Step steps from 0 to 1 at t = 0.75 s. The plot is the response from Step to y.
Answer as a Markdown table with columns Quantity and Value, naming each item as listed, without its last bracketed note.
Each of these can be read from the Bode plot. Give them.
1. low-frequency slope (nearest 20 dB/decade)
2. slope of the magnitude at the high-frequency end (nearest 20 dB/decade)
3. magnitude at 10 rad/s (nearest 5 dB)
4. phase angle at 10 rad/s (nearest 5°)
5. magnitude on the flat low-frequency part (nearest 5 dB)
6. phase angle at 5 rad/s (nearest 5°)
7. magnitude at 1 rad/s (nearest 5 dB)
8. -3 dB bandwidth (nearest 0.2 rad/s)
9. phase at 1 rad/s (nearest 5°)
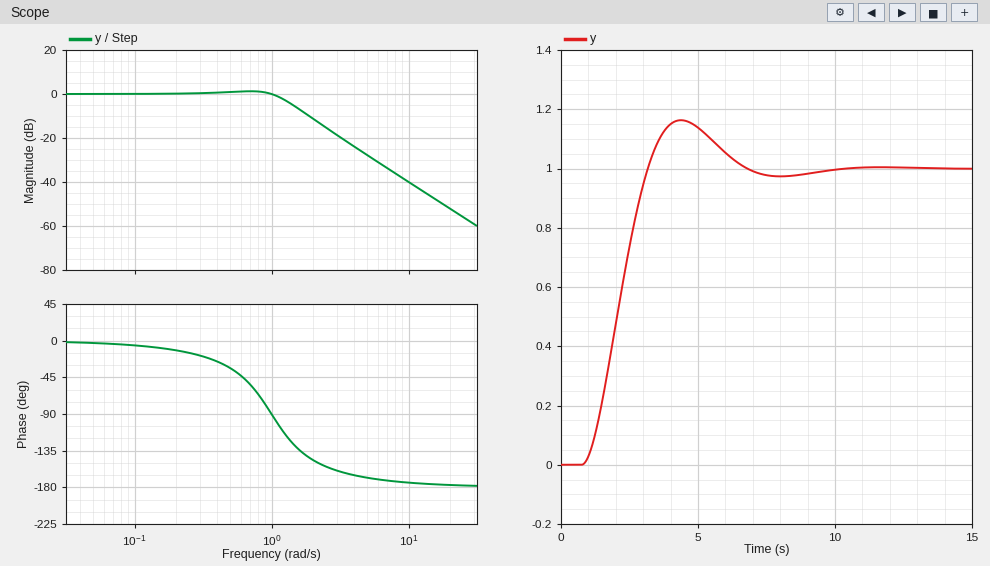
| Quantity | Value |
|---|---|
| low-frequency slope | 0 dB/decade |
| slope of the magnitude at the high-frequency end | -40 dB/decade |
| magnitude at 10 rad/s | -40 dB |
| phase angle at 10 rad/s | -175° |
| magnitude on the flat low-frequency part | 0 dB |
| phase angle at 5 rad/s | -170° |
| magnitude at 1 rad/s | 0 dB |
| -3 dB bandwidth | 1.2 rad/s |
| phase at 1 rad/s | -90° |
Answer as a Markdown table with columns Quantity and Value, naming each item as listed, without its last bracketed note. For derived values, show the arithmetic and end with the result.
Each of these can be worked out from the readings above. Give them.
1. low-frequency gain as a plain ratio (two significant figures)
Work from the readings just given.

| Quantity | Value |
|---|---|
| low-frequency gain as a plain ratio | 10^(0 / 20) = 1.0 |
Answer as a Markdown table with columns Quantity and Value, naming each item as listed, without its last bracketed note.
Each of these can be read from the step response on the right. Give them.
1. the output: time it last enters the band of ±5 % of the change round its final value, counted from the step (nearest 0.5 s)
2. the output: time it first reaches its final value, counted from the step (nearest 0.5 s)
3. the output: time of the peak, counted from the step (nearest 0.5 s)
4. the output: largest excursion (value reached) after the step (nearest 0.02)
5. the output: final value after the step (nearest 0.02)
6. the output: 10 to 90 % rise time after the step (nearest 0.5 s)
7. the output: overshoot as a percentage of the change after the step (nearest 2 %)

| Quantity | Value |
|---|---|
| the output: time it last enters the band of ±5 % of the change round its final value, counted from the step | 5.5 s |
| the output: time it first reaches its final value, counted from the step | 2.5 s |
| the output: time of the peak, counted from the step | 3.5 s |
| the output: largest excursion (value reached) after the step | 1.16 |
| the output: final value after the step | 1.00 |
| the output: 10 to 90 % rise time after the step | 1.5 s |
| the output: overshoot as a percentage of the change after the step | 16 % |
